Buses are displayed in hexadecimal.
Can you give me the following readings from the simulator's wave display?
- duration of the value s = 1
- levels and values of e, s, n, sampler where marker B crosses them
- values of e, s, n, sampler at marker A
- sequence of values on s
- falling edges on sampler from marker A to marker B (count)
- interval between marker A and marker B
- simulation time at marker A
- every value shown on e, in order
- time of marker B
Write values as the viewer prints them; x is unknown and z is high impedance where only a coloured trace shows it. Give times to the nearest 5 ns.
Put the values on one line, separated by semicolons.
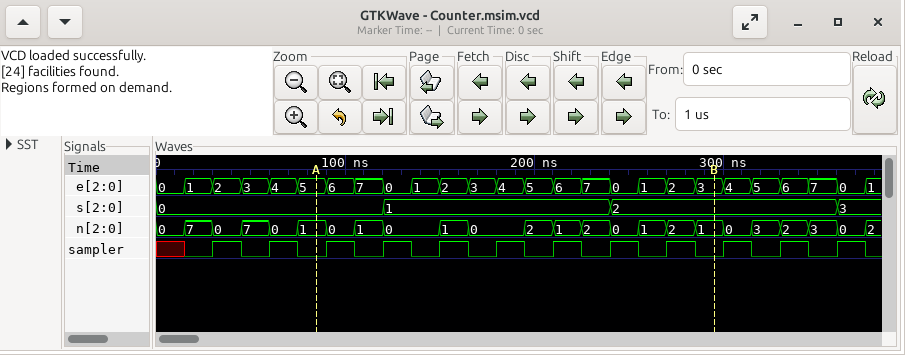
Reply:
120 ns; e=3, s=2, n=1, sampler=0; e=5, s=0, n=1, sampler=0; 0, 1, 2, 3; 7; 210 ns; 85 ns; 0, 1, 2, 3, 4, 5, 6, 7, 0, 1, 2, 3, 4, 5, 6, 7, 0, 1, 2, 3, 4, 5, 6, 7, 0, 1; 295 ns
